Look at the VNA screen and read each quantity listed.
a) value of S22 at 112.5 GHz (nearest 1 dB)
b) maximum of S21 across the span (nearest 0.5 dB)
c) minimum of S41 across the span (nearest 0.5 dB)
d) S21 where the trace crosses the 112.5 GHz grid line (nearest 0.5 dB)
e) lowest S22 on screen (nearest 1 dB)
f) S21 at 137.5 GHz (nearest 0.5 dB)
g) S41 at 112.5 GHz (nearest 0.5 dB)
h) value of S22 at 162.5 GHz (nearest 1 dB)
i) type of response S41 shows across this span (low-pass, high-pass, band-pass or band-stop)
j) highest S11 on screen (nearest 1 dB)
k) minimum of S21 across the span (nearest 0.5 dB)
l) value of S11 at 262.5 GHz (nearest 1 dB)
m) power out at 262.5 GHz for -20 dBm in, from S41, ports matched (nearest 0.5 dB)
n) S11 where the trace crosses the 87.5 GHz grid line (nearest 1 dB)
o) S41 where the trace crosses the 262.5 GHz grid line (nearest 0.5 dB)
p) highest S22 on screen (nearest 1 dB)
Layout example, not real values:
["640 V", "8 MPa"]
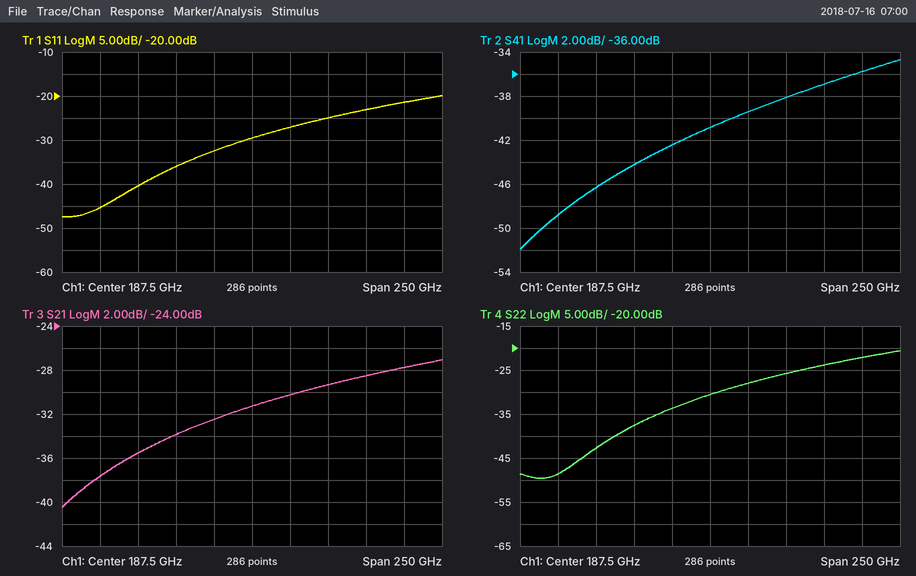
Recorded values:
["-43 dB", "-27.0 dB", "-52.0 dB", "-35.5 dB", "-50 dB", "-34.0 dB", "-46.5 dB", "-34 dB", "high-pass", "-20 dB", "-40.5 dB", "-23 dB", "-57.0 dBm", "-45 dB", "-37.0 dB", "-21 dB"]
